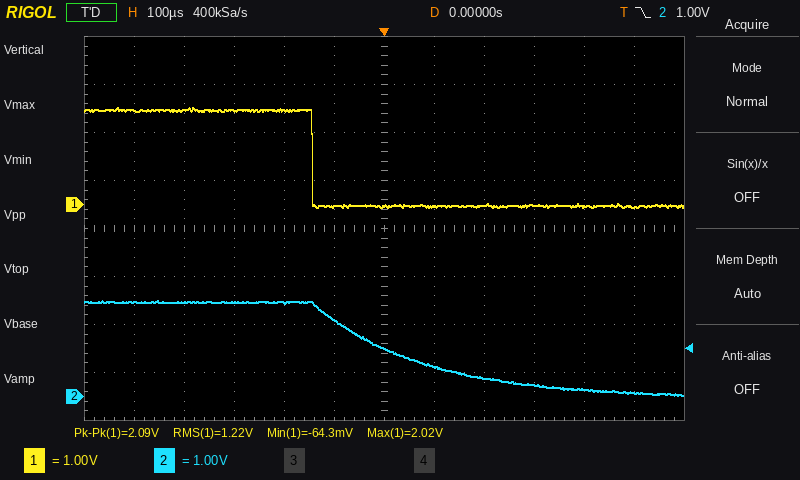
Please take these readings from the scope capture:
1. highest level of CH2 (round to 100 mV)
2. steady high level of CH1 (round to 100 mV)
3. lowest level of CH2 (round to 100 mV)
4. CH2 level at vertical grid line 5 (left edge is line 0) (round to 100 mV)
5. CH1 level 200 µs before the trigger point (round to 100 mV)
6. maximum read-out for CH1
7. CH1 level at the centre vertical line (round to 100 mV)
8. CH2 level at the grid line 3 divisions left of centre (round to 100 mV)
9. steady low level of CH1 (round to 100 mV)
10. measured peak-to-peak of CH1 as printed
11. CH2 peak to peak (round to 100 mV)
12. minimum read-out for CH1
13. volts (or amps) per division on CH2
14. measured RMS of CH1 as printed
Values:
2.0 V
2.0 V
0.0 V
1.6 V
2.0 V
2.02 V
0.0 V
2.0 V
0.0 V
2.09 V
2.0 V
-64.3 mV
1 V
1.22 V
